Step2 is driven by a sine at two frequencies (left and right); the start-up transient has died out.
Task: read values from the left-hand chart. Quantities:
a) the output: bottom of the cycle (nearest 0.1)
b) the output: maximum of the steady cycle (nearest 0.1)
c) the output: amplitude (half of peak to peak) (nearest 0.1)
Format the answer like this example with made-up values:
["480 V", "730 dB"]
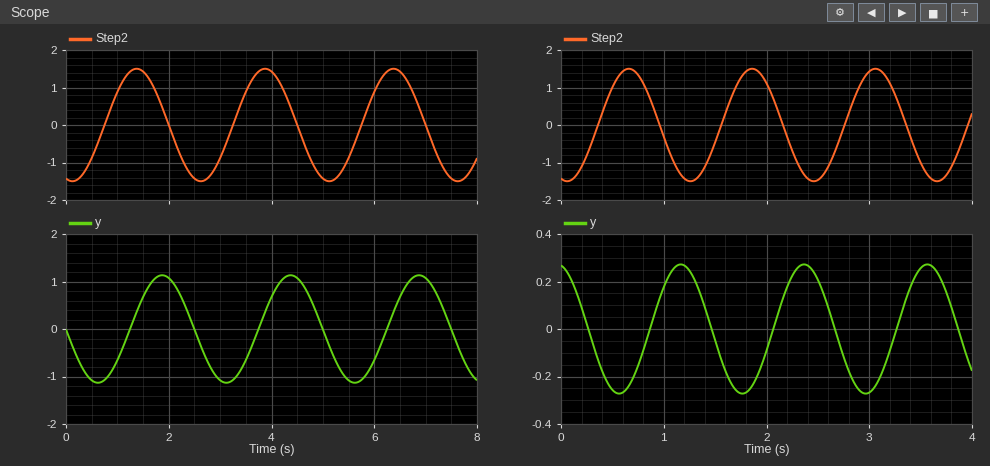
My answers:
["-1.1", "1.1", "1.1"]
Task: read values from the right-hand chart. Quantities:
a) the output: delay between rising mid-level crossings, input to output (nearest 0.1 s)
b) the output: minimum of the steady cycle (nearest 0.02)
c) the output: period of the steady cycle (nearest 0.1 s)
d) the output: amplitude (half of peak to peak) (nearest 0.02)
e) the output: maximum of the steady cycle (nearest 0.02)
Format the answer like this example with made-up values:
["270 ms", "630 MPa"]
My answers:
["0.5 s", "-0.28", "1.2 s", "0.28", "0.28"]
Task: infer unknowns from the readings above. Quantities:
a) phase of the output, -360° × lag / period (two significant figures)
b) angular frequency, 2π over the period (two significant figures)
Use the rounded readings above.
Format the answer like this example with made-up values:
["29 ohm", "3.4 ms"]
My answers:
["-150°", "5.2 rad/s"]
